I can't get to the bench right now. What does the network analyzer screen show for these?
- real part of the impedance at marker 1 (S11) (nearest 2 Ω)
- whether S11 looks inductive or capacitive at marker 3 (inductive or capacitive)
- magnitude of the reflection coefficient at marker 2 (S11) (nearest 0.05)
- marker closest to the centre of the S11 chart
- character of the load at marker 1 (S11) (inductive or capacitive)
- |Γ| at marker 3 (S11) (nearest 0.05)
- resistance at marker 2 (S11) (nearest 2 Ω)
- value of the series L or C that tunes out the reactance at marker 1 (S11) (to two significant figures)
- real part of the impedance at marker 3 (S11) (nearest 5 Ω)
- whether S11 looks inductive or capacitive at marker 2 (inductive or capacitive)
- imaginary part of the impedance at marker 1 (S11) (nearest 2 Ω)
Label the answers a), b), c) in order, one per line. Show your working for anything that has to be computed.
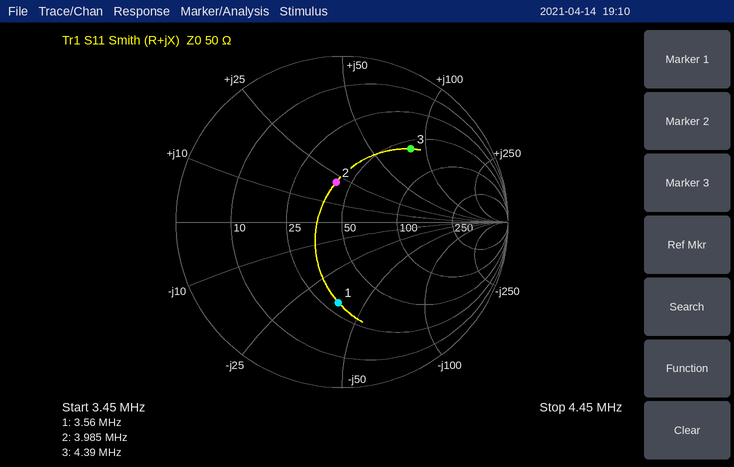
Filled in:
a) 30 Ω
b) inductive
c) 0.25
d) marker 2
e) capacitive
f) 0.60
g) 42 Ω
h) L = 38 Ω/(2π × 3.56 MHz) ≈ 1.7 µH
i) 60 Ω
j) inductive
k) -38 Ω
